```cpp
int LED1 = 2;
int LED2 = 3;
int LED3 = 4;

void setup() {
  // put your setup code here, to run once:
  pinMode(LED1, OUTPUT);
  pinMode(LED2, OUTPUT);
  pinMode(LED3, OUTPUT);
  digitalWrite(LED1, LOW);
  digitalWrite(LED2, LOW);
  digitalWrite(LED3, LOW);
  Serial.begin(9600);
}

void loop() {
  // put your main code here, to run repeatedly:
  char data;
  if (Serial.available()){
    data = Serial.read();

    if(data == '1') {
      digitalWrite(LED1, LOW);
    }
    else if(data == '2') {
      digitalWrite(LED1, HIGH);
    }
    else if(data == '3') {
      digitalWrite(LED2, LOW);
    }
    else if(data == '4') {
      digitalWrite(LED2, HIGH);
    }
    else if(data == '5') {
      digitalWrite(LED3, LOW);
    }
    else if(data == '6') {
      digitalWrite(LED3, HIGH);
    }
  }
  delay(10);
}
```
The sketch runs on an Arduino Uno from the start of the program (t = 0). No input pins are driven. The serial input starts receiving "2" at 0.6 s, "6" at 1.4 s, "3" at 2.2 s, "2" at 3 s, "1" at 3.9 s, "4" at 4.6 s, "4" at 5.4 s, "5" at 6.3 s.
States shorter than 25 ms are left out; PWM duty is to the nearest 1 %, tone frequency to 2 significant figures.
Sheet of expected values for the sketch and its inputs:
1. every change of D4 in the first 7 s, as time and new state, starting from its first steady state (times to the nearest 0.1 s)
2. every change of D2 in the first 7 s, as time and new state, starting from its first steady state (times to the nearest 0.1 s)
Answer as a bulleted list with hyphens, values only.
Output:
- 0 s low; 1.4 s high; 6.3 s low
- 0 s low; 0.6 s high; 3.9 s low
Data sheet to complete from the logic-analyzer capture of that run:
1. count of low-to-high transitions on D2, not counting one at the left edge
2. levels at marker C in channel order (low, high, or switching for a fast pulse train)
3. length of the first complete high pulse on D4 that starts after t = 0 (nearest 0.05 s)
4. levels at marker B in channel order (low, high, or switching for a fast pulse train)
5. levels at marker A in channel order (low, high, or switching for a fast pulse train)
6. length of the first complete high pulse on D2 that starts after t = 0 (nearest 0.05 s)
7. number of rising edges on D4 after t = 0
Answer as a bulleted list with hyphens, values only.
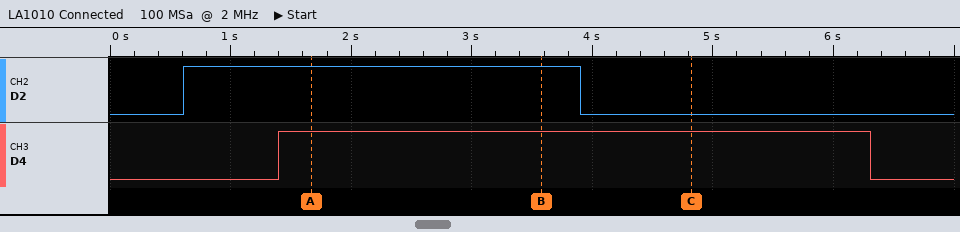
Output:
- 1
- D2 low, D4 high
- 4.90 s
- D2 high, D4 high
- D2 high, D4 high
- 3.30 s
- 1
